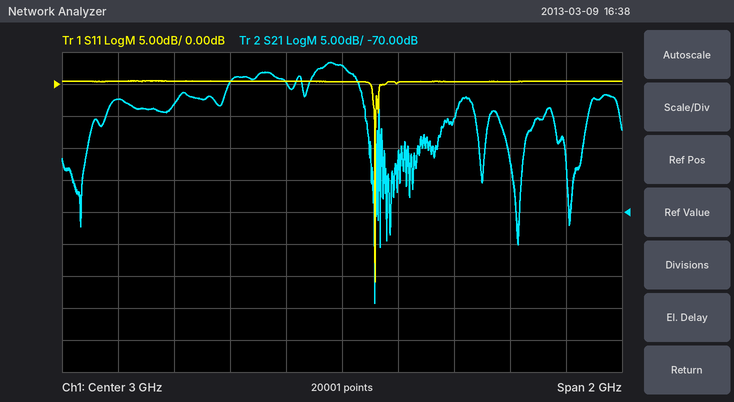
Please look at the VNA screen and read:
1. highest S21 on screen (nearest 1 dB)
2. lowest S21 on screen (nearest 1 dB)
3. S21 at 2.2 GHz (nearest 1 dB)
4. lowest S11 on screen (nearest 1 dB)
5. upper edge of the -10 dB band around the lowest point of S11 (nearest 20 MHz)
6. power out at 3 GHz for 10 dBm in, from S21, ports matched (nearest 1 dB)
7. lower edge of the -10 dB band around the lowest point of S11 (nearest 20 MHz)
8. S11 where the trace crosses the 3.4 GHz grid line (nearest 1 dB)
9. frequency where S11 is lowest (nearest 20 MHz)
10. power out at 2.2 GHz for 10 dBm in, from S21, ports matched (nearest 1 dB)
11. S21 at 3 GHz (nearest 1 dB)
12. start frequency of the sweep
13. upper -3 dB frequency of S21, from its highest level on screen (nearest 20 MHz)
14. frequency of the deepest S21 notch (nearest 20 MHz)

-47 dB
-84 dB
-52 dB
-31 dB
3.12 GHz
-37 dBm
3.12 GHz
0 dB
3.12 GHz
-42 dBm
-47 dB
2 GHz
3.06 GHz
3.12 GHz
